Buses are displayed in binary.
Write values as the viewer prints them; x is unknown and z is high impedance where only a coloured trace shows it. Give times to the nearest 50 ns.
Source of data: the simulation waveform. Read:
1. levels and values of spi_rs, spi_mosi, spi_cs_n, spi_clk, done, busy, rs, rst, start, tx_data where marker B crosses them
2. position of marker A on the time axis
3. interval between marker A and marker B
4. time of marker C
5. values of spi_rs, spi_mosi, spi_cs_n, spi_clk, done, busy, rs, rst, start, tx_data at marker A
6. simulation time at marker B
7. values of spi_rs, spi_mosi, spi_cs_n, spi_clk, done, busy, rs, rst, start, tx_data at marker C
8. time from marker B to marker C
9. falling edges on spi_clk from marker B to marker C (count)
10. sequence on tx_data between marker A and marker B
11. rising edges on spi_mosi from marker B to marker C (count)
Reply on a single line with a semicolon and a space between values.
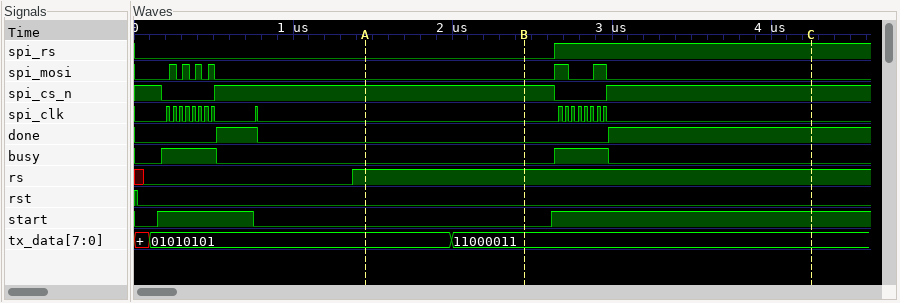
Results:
spi_rs=0, spi_mosi=0, spi_cs_n=1, spi_clk=0, done=0, busy=0, rs=1, rst=0, start=0, tx_data=11000011; 1450 ns; 1000 ns; 4250 ns; spi_rs=0, spi_mosi=0, spi_cs_n=1, spi_clk=0, done=0, busy=0, rs=1, rst=0, start=0, tx_data=01010101; 2450 ns; spi_rs=1, spi_mosi=0, spi_cs_n=1, spi_clk=0, done=1, busy=0, rs=1, rst=0, start=1, tx_data=11000011; 1800 ns; 8; 01010101, 11000011; 2
